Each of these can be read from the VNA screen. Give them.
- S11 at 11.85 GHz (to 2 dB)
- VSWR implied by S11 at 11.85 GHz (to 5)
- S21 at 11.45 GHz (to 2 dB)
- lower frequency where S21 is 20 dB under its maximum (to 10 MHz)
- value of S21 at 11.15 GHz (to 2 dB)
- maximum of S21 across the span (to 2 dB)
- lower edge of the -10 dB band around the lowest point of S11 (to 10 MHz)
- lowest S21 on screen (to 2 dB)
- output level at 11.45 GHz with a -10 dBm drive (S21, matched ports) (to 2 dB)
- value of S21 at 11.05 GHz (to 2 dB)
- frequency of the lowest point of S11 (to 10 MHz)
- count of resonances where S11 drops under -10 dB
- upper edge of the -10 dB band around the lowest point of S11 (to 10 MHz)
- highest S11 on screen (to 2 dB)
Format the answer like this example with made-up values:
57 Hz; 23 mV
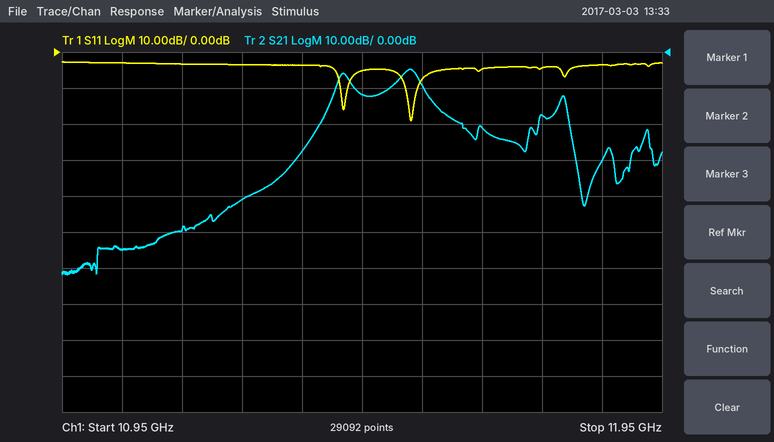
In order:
-4 dB; 5; -12 dB; 11.36 GHz; -50 dB; -4 dB; 11.52 GHz; -62 dB; -22 dBm; -54 dB; 11.53 GHz; 2; 11.54 GHz; -2 dB
